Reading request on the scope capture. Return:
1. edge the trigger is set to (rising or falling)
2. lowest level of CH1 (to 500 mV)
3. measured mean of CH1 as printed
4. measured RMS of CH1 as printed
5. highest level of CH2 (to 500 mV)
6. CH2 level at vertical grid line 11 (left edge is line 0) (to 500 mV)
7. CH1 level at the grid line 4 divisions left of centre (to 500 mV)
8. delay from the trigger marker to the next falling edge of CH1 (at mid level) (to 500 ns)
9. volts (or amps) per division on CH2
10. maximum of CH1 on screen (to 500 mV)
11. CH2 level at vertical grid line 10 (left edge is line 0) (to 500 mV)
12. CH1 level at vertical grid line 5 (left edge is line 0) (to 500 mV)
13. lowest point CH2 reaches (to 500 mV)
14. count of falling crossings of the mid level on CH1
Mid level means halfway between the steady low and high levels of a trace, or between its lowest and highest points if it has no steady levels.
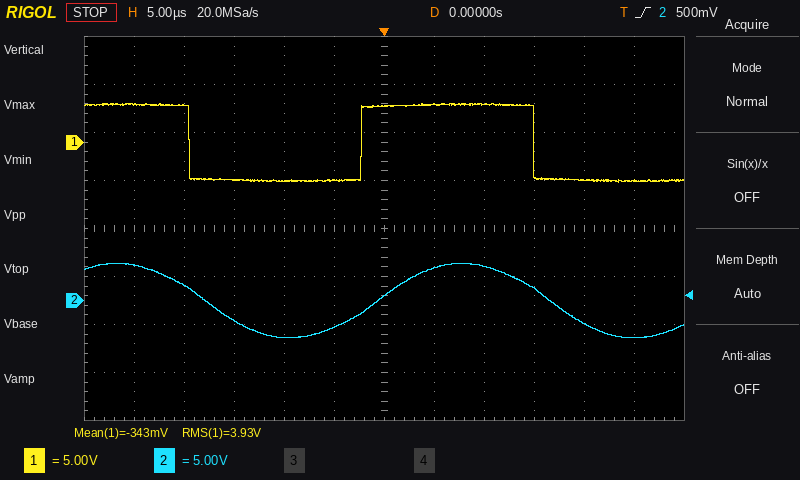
rising
-4.0 V
-343 mV
3.93 V
4.0 V
-4.0 V
4.0 V
15.0 µs
5 V
4.0 V
-2.5 V
-4.0 V
-4.0 V
2
